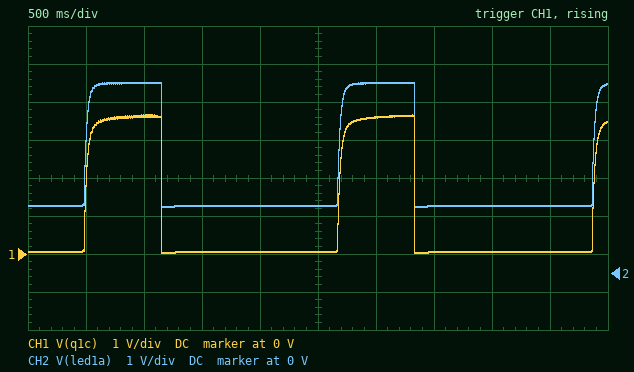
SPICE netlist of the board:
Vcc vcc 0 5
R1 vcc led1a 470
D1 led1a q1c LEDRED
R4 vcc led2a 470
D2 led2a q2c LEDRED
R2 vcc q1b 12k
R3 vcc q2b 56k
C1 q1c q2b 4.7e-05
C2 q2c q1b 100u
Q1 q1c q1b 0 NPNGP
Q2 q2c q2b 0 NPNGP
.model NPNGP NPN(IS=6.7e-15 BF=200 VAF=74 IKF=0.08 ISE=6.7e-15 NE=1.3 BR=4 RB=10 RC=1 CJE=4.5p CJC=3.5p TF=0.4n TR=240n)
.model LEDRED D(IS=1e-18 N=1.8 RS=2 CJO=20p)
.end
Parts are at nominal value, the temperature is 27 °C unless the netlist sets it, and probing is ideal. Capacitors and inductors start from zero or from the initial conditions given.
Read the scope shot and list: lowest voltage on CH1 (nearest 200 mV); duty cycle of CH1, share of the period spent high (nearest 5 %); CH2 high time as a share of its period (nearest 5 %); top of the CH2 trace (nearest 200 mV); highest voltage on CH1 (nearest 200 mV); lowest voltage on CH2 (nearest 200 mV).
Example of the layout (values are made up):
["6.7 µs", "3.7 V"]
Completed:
["0 V", "30 %", "30 %", "5.0 V", "3.6 V", "1.8 V"]
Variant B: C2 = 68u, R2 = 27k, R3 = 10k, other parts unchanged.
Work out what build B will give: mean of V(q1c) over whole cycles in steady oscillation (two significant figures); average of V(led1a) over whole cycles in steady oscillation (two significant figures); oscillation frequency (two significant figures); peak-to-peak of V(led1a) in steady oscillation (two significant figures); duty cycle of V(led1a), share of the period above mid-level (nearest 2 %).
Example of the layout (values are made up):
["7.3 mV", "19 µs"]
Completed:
["2.8 V", "4.3 V", "760 mHz", "3.3 V", "78 %"]
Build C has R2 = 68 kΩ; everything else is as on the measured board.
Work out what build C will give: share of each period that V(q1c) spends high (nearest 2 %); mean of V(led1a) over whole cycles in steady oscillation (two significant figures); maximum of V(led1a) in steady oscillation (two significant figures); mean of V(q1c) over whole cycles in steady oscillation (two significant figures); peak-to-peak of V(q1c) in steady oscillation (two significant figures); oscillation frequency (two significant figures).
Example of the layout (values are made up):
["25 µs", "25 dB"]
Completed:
["72 %", "4.1 V", "5.0 V", "2.7 V", "3.7 V", "190 mHz"]
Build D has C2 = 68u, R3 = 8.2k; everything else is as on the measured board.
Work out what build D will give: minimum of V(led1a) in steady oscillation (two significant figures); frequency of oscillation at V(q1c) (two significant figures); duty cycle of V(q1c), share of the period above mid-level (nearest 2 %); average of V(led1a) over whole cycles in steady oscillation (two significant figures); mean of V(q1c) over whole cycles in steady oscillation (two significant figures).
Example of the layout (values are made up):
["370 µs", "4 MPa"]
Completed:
["1.7 V", "1.5 Hz", "66 %", "3.8 V", "2.3 V"]
